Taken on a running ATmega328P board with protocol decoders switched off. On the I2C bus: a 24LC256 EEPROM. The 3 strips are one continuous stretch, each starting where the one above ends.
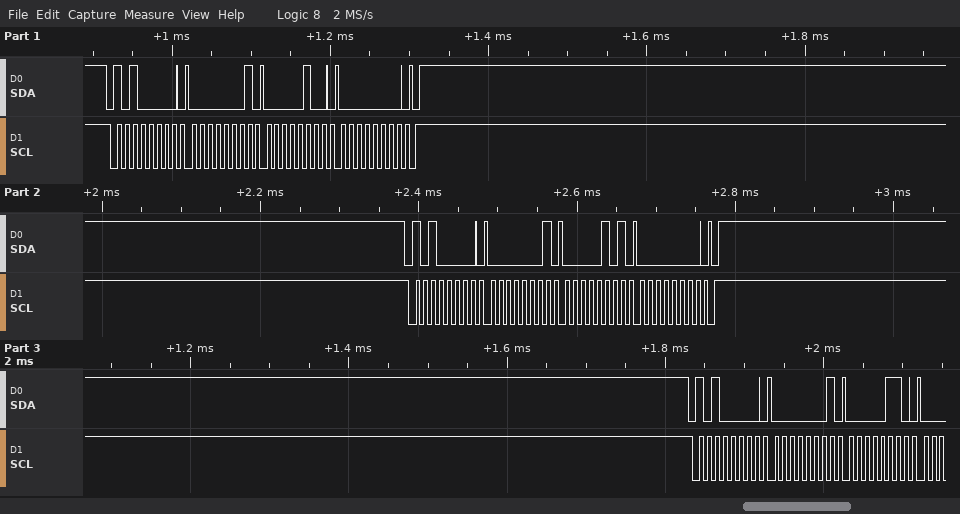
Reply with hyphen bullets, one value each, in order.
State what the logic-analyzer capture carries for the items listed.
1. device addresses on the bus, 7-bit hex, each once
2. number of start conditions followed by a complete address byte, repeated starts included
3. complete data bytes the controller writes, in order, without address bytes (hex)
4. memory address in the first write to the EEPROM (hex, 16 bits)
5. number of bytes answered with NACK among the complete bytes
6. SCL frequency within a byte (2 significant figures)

- 0x50
- 3
- 01 04 00 01 05 00 01 06
- 0x0104
- 0
- 100 kHz
